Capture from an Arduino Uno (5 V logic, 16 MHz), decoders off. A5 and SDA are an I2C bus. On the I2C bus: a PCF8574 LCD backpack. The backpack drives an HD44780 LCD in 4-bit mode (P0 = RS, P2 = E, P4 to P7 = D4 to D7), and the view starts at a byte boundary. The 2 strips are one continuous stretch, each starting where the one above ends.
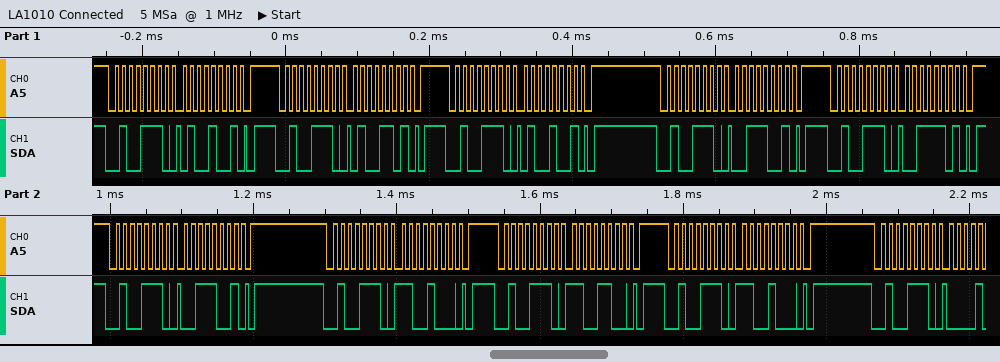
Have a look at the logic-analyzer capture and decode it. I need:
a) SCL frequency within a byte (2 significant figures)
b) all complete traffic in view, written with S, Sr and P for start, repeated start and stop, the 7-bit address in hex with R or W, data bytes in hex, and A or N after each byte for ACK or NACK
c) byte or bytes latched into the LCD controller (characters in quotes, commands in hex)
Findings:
100 kHz
S 27W A 49 A P S 27W A 4D A P S 27W A 49 A P S 27W A 39 A P S 27W A 3D A P S 27W A 39 A P S 27W A C8 A P S 27W A CC A P S 27W A C8 A P S 27W A
'C'
